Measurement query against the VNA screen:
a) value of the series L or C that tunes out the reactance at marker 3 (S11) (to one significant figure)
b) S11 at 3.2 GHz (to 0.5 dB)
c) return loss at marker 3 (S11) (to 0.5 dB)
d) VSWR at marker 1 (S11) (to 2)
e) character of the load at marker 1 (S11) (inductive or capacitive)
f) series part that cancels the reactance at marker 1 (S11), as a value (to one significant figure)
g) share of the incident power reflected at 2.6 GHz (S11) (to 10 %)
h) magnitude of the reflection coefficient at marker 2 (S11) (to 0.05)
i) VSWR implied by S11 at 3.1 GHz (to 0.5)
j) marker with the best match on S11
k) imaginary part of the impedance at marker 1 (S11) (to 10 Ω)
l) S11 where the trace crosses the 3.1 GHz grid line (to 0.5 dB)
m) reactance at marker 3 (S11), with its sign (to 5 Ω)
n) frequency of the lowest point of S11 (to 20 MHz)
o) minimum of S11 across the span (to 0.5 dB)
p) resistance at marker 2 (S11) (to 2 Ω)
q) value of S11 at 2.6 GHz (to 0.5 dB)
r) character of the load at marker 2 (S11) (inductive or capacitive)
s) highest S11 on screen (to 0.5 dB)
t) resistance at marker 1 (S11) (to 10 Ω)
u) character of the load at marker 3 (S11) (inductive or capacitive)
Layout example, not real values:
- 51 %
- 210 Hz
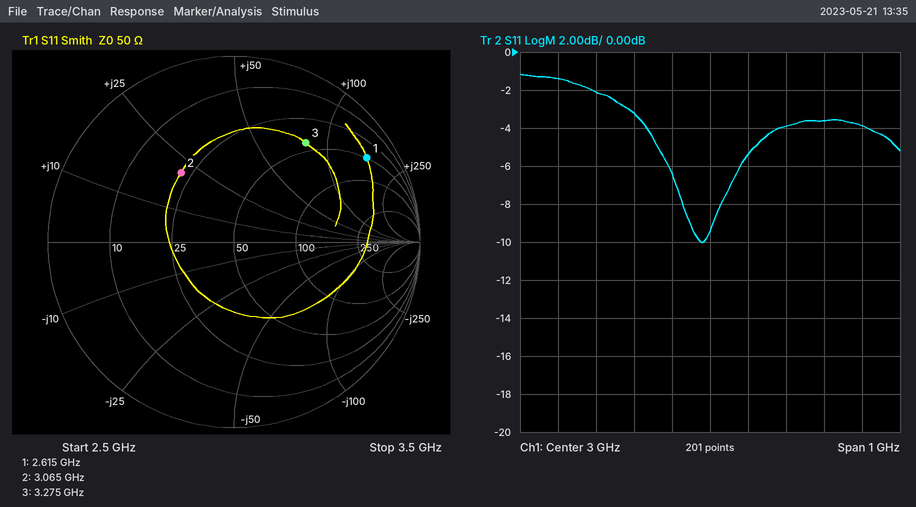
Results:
- 600 fF
- -4.0 dB
- 3.5 dB
- 12
- inductive
- 400 fF
- 70 %
- 0.45
- 3.5
- marker 2
- +160 Ω
- -5.5 dB
- +80 Ω
- 2.98 GHz
- -10.0 dB
- 22 Ω
- -1.5 dB
- inductive
- -1.0 dB
- 50 Ω
- inductive
